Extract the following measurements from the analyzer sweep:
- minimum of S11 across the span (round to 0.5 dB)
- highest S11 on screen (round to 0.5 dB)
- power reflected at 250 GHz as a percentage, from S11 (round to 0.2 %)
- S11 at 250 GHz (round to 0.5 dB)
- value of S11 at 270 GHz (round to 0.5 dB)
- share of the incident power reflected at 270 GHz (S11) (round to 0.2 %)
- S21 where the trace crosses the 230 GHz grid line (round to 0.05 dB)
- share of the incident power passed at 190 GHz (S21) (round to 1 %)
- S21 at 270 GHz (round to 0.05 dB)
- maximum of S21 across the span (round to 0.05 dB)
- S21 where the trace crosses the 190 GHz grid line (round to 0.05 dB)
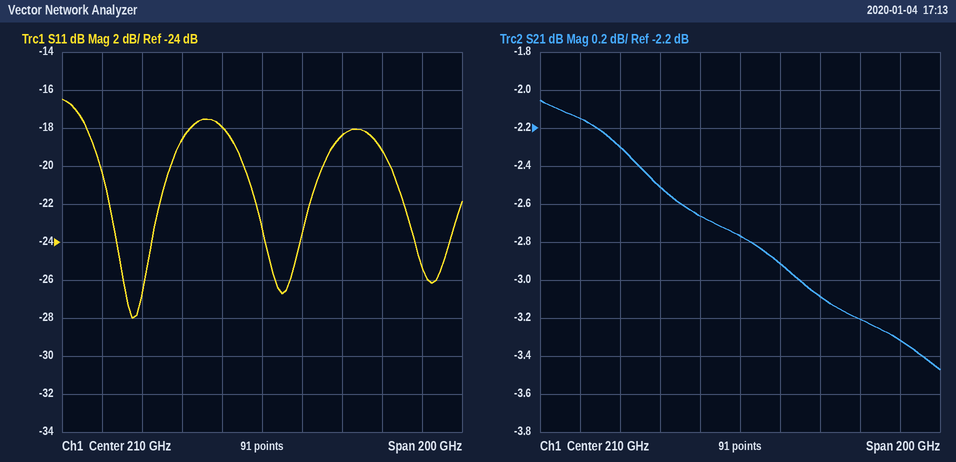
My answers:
-28.0 dB
-16.5 dB
1.4 %
-18.5 dB
-19.0 dB
1.2 %
-2.90 dB
54 %
-3.20 dB
-2.05 dB
-2.65 dB
